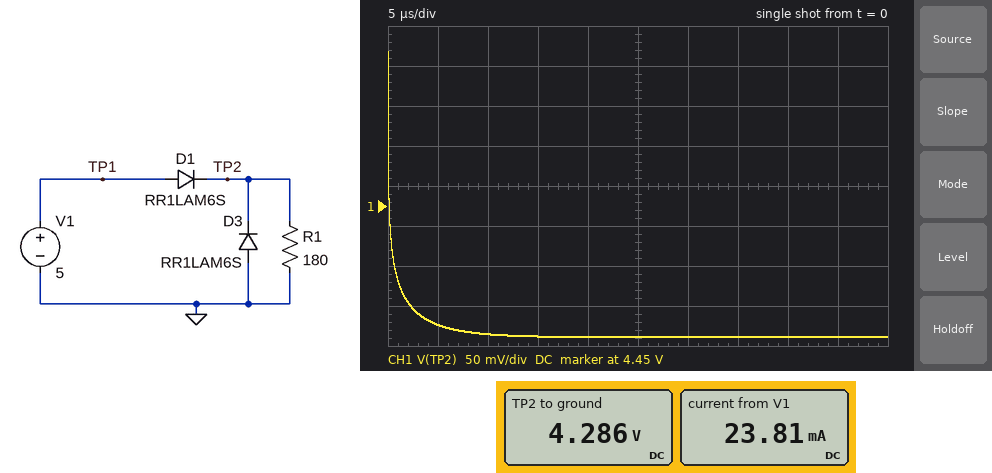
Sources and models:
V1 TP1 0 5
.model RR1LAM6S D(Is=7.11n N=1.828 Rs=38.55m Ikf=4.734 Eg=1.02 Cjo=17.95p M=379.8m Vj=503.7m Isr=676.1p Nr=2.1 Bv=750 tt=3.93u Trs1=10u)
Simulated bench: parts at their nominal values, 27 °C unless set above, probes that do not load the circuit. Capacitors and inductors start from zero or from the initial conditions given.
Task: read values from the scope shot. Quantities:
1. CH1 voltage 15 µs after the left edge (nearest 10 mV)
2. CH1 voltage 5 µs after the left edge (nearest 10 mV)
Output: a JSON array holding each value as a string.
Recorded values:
["4.29 V", "4.30 V"]
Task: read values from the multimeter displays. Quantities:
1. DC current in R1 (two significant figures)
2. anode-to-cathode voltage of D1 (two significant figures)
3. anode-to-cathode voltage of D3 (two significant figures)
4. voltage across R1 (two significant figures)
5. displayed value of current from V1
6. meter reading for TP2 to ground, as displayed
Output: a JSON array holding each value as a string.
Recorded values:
["24 mA", "710 mV", "-4.3 V", "4.3 V", "23.81 mA", "4.286 V"]
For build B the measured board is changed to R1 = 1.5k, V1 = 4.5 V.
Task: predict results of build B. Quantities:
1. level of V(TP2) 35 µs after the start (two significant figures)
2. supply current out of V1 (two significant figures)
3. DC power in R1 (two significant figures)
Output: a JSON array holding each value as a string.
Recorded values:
["3.9 V", "2.6 mA", "10 mW"]
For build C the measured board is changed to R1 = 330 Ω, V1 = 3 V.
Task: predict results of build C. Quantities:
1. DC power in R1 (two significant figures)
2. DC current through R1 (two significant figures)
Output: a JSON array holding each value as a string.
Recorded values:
["17 mW", "7.1 mA"]
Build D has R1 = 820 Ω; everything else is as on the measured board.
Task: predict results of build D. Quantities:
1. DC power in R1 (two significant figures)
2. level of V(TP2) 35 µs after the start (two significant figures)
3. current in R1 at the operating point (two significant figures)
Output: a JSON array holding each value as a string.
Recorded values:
["23 mW", "4.4 V", "5.3 mA"]
